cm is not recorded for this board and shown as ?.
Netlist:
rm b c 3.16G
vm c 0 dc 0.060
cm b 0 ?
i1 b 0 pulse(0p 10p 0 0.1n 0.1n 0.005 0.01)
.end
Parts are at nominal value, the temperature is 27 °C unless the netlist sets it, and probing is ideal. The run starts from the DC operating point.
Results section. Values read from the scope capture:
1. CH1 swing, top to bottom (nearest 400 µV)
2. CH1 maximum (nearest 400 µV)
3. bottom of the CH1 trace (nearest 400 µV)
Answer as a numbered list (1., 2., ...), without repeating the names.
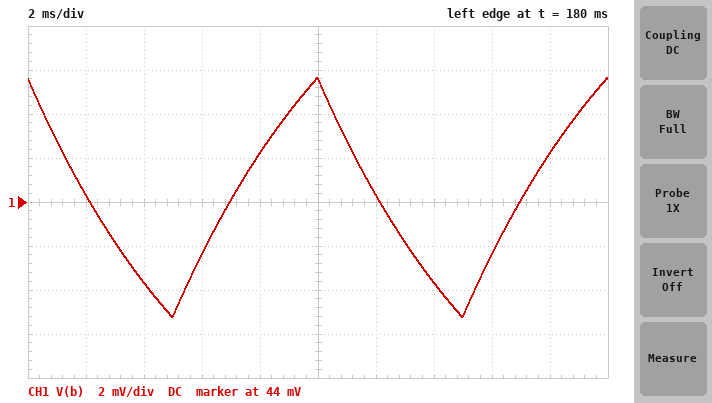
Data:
1. 10.8 mV
2. 49.6 mV
3. 38.8 mV
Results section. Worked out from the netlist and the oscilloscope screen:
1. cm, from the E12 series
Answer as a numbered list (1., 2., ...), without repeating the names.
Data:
1. 2.2 pF
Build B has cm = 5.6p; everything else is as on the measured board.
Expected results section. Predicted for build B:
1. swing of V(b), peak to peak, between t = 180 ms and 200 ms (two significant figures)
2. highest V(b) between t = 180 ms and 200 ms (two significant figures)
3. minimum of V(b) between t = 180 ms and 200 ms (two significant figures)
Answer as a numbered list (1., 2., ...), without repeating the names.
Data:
1. 4.4 mV
2. 46 mV
3. 42 mV
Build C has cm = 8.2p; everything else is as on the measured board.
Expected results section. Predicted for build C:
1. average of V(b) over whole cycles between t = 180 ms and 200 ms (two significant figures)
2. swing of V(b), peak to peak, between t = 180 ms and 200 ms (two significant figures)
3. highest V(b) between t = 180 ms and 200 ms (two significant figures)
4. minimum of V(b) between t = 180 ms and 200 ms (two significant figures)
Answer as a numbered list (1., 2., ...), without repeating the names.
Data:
1. 44 mV
2. 3.0 mV
3. 46 mV
4. 43 mV
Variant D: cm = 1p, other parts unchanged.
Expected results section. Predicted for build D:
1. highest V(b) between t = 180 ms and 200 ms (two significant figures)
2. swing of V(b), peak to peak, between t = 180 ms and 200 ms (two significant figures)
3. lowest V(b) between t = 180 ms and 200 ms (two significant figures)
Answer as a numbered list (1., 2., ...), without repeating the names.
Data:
1. 55 mV
2. 21 mV
3. 34 mV
